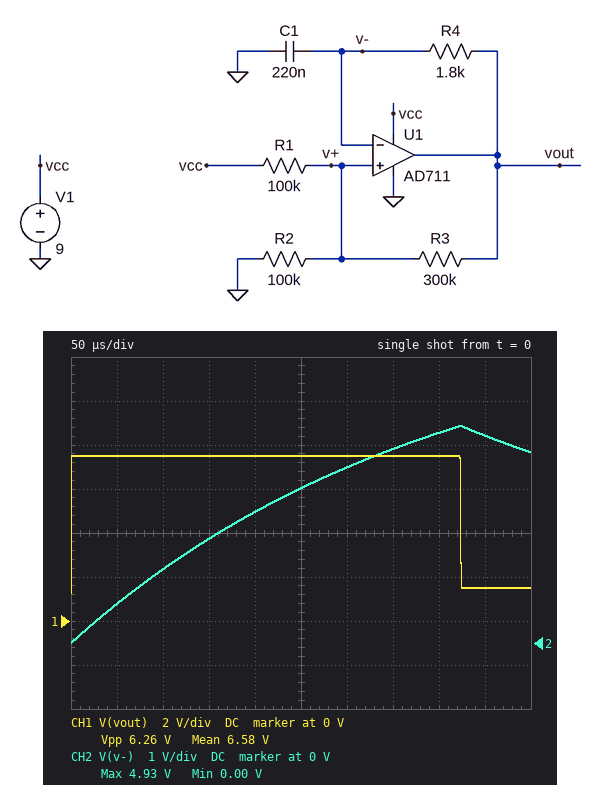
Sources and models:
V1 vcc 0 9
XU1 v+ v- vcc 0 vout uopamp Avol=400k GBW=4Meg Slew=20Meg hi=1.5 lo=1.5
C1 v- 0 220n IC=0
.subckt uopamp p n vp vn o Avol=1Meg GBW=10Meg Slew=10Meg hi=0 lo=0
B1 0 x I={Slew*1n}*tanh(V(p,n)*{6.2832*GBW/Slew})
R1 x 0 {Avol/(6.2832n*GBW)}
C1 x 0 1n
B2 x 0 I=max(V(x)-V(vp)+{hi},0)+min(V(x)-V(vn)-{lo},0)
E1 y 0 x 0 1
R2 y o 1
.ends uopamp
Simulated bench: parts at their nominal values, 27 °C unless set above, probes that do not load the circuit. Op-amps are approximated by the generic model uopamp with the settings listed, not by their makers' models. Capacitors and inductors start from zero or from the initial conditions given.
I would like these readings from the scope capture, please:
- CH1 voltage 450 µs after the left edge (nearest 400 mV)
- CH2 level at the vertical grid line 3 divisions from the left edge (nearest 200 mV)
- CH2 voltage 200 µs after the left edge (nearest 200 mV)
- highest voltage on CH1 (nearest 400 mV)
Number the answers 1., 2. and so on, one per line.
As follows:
1. 1.6 V
2. 2.4 V
3. 3.0 V
4. 7.6 V
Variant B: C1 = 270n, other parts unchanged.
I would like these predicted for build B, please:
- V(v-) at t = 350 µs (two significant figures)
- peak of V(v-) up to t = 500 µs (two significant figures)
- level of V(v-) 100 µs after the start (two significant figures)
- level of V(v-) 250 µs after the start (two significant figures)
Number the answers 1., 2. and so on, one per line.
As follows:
1. 3.9 V
2. 4.8 V
3. 1.4 V
4. 3.0 V
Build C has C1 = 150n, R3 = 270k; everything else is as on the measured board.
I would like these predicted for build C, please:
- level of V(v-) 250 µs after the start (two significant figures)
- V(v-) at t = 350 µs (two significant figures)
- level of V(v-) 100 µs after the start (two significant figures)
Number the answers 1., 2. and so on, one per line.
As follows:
1. 4.5 V
2. 4.3 V
3. 2.3 V
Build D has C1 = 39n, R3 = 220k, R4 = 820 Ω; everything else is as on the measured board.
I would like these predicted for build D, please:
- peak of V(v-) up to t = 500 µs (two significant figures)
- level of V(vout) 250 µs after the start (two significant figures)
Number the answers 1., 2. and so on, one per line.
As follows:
1. 5.1 V
2. 1.5 V
